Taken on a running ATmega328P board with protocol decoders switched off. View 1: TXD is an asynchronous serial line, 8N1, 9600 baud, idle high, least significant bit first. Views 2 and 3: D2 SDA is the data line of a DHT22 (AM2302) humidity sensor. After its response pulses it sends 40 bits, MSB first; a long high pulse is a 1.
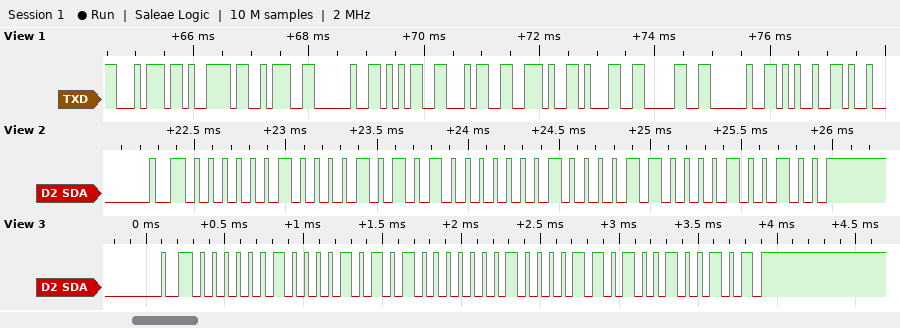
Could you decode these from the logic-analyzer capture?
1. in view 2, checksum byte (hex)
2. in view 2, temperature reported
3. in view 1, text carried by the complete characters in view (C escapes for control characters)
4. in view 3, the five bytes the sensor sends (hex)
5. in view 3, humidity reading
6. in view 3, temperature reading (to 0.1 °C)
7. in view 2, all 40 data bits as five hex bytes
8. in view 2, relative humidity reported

0x24
26.8 °C
"ty: 54.10 %"
02 15 01 0D 25
53.3 %
26.9 °C
02 15 01 0C 24
53.3 %
